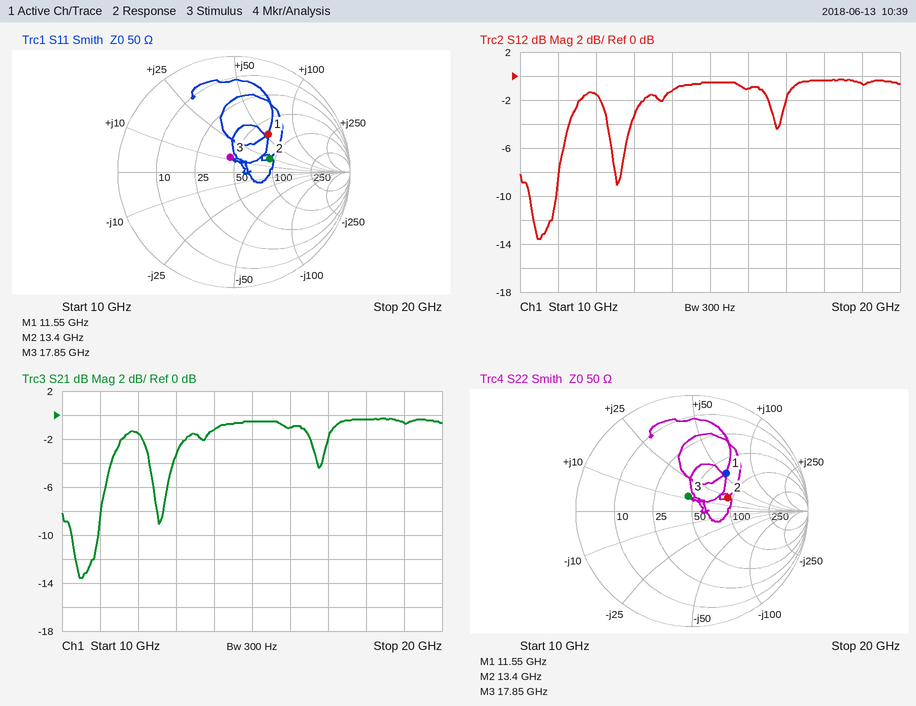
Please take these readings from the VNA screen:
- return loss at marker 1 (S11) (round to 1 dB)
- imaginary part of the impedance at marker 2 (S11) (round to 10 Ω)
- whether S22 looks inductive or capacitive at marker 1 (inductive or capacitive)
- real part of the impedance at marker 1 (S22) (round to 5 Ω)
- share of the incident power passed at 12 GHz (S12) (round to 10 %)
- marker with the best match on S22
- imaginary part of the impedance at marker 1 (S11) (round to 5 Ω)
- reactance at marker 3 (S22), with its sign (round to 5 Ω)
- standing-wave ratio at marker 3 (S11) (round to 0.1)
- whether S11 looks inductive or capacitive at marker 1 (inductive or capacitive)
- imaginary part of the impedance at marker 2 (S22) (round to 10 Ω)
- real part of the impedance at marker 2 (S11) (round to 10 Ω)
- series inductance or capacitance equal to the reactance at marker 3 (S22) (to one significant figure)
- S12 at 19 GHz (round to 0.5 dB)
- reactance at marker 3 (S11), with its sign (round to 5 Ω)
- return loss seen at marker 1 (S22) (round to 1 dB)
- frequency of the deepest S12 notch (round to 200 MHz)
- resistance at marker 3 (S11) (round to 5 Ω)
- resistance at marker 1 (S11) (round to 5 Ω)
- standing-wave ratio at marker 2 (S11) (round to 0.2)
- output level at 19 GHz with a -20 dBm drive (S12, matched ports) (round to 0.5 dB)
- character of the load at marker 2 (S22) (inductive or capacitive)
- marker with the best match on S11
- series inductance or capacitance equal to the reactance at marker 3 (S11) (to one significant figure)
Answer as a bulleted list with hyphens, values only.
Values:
- 7 dB
- +20 Ω
- inductive
- 65 Ω
- 70 %
- marker 3
- +55 Ω
- +10 Ω
- 1.3
- inductive
- +20 Ω
- 90 Ω
- 100 pH
- -0.5 dB
- +10 Ω
- 7 dB
- 10.4 GHz
- 45 Ω
- 65 Ω
- 2.0
- -20.5 dBm
- inductive
- marker 3
- 100 pH
